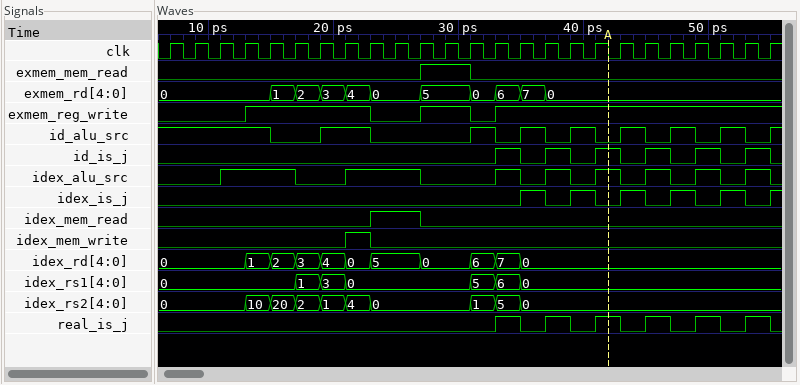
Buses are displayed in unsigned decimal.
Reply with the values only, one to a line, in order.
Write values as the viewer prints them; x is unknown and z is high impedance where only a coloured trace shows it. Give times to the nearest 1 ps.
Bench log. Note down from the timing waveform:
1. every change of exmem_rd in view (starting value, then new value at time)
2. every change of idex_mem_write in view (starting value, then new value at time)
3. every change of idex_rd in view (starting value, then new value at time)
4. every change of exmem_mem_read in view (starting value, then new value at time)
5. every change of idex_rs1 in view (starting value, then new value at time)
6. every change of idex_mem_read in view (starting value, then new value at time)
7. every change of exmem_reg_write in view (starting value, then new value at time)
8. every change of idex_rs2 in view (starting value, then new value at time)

0, 1 at 15 ps, 2 at 17 ps, 3 at 19 ps, 4 at 21 ps, 0 at 23 ps, 5 at 27 ps, 0 at 31 ps, 6 at 33 ps, 7 at 35 ps, 0 at 37 ps
0, 1 at 21 ps, 0 at 23 ps
0, 1 at 13 ps, 2 at 15 ps, 3 at 17 ps, 4 at 19 ps, 0 at 21 ps, 5 at 23 ps, 0 at 27 ps, 6 at 31 ps, 7 at 33 ps, 0 at 35 ps
0, 1 at 27 ps, 0 at 31 ps
0, 1 at 17 ps, 3 at 19 ps, 0 at 21 ps, 5 at 31 ps, 6 at 33 ps, 0 at 35 ps
0, 1 at 23 ps, 0 at 27 ps
0, 1 at 13 ps, 0 at 23 ps, 1 at 27 ps, 0 at 31 ps, 1 at 33 ps
0, 10 at 13 ps, 20 at 15 ps, 2 at 17 ps, 1 at 19 ps, 4 at 21 ps, 0 at 23 ps, 1 at 31 ps, 5 at 33 ps, 0 at 35 ps
